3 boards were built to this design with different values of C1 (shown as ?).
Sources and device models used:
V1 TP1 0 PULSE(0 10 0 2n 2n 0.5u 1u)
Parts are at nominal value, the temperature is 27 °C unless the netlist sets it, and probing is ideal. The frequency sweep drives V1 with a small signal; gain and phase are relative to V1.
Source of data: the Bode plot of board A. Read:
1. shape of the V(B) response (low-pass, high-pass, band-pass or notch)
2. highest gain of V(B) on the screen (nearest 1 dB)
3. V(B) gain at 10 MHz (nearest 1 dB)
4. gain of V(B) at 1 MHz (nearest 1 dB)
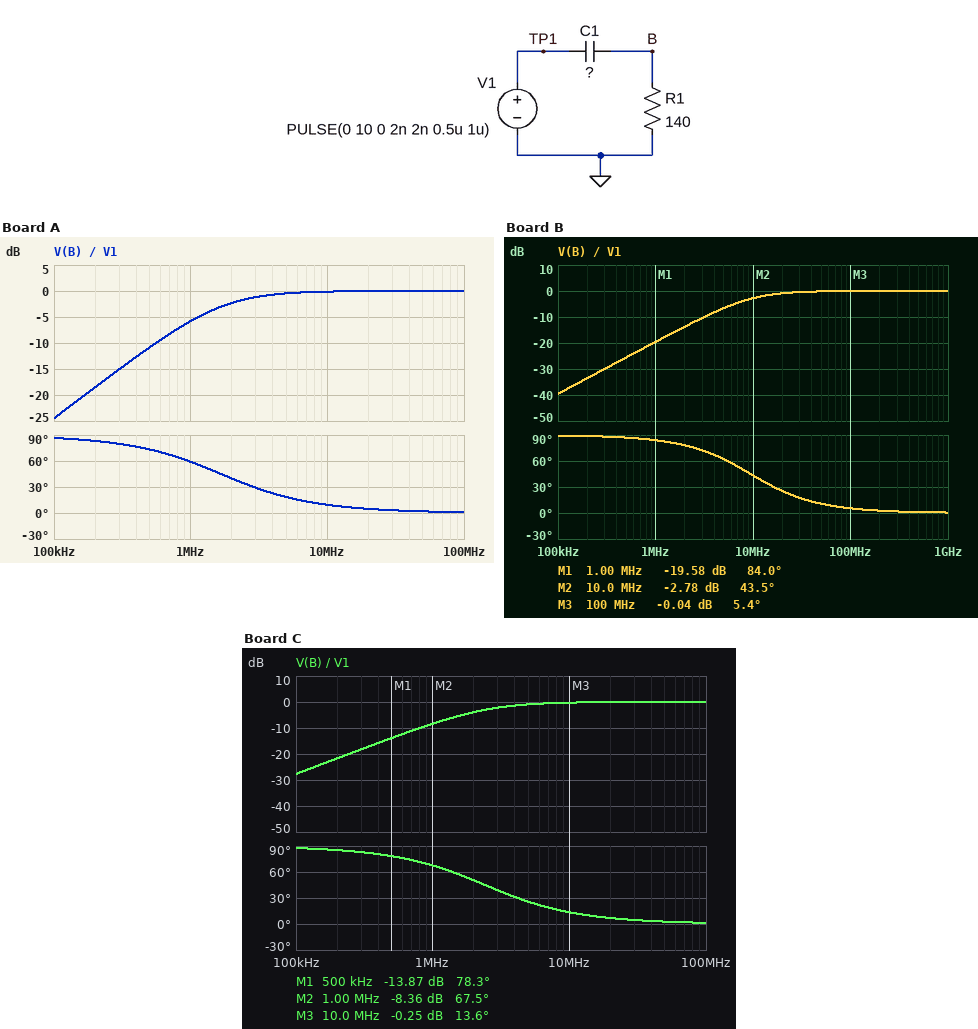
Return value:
high-pass
0 dB
0 dB
-6 dB
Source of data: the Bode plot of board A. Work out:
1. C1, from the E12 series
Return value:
680 pF
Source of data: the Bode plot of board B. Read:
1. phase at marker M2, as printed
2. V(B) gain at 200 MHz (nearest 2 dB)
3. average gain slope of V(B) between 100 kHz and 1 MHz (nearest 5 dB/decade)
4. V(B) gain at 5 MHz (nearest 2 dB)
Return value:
43.5 deg
0 dB
20 dB/decade
-6 dB
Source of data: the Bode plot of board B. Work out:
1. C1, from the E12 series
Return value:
120 pF
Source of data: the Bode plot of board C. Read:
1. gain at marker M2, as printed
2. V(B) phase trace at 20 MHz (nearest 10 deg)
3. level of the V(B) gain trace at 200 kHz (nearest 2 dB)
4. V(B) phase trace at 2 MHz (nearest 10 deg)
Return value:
-8.36 dB
10 deg
-22 dB
50 deg
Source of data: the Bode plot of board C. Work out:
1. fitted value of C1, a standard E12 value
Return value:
470 pF
